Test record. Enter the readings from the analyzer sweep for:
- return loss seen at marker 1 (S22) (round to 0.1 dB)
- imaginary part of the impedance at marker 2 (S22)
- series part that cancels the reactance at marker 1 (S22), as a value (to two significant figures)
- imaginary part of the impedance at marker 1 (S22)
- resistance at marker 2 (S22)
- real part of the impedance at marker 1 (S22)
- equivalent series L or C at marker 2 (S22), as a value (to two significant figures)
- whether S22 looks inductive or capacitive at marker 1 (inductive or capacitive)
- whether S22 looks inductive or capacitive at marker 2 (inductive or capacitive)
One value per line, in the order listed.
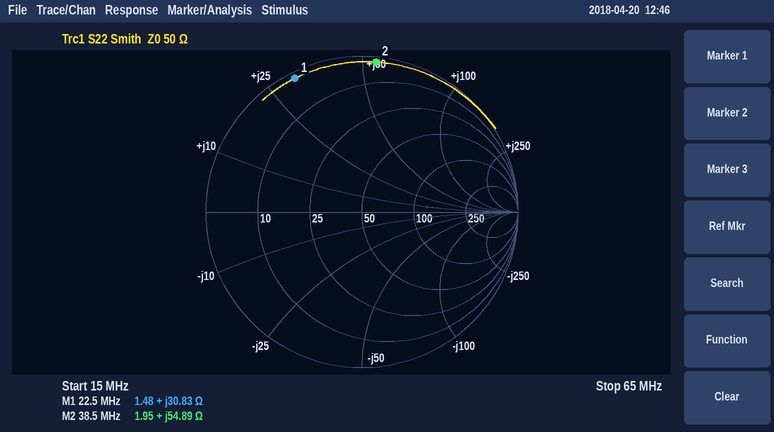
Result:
0.4 dB
+54.89 Ω
230 pF
+30.83 Ω
1.95 Ω
1.48 Ω
230 nH
inductive
inductive
